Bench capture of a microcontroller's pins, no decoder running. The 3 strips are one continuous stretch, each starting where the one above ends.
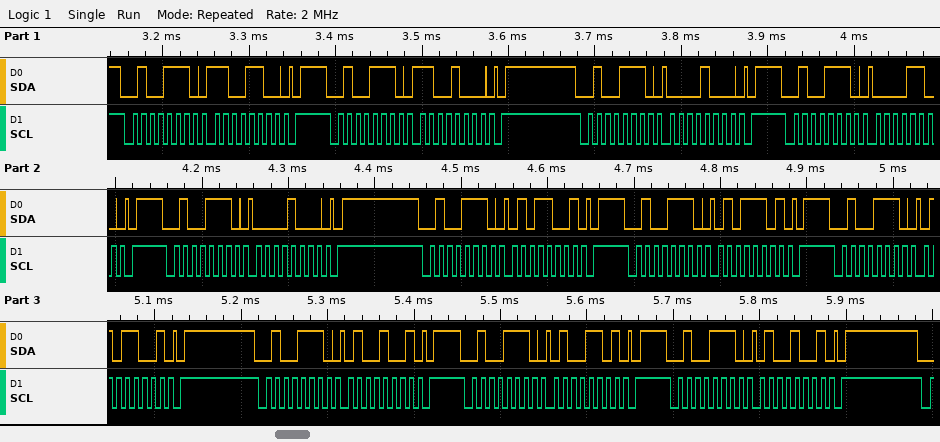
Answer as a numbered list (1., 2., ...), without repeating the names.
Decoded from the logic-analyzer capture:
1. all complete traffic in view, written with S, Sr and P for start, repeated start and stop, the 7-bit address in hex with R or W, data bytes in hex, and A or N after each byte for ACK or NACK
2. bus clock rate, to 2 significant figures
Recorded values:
1. S 27W A CC A P S 27W A C8 A P S 27W A 08 A P S 27W A 0C A P S 27W A 08 A P S 27W A 59 A P S 27W A 5D A P S 27W A 59 A P S 27W A 49 A P S 27W A 4D A P S 27W A 49 A P
2. 100 kHz
